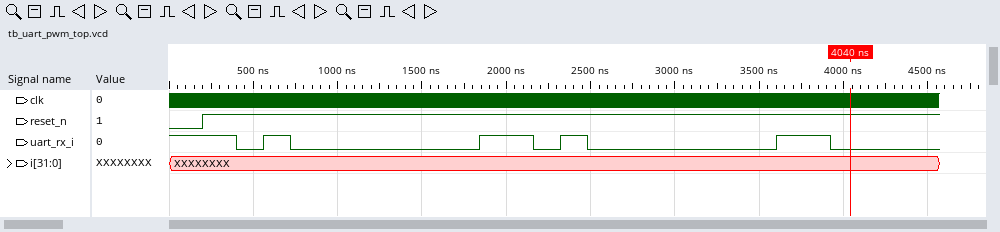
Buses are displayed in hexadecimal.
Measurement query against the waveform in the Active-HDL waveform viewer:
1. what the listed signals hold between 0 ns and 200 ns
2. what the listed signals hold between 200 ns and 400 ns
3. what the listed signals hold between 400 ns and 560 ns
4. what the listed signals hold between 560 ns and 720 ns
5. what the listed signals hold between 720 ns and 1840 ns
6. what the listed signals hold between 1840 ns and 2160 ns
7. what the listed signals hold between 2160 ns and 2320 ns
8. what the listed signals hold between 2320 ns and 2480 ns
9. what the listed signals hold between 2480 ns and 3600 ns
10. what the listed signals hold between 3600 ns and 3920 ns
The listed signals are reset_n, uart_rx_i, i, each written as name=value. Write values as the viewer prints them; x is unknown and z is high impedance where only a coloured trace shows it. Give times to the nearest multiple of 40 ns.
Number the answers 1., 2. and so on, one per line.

1. reset_n=0, uart_rx_i=1, i=XXXXXXXX
2. reset_n=1, uart_rx_i=1, i=XXXXXXXX
3. reset_n=1, uart_rx_i=0, i=XXXXXXXX
4. reset_n=1, uart_rx_i=1, i=XXXXXXXX
5. reset_n=1, uart_rx_i=0, i=XXXXXXXX
6. reset_n=1, uart_rx_i=1, i=XXXXXXXX
7. reset_n=1, uart_rx_i=0, i=XXXXXXXX
8. reset_n=1, uart_rx_i=1, i=XXXXXXXX
9. reset_n=1, uart_rx_i=0, i=XXXXXXXX
10. reset_n=1, uart_rx_i=1, i=XXXXXXXX
